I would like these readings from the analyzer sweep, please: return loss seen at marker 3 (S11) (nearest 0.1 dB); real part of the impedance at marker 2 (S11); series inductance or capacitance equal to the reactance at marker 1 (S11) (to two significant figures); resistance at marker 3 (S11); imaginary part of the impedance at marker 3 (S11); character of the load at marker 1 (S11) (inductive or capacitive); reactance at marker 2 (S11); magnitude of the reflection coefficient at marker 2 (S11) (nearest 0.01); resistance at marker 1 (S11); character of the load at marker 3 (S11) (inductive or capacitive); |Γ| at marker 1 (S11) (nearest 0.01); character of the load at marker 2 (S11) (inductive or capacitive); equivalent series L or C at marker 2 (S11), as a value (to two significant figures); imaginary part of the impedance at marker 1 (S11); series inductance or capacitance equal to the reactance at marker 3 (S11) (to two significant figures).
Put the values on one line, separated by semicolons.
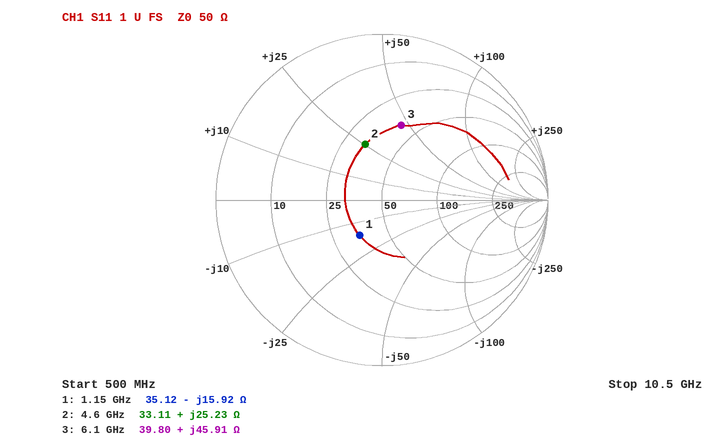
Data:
6.6 dB; 33.11 Ω; 8.7 pF; 39.80 Ω; +45.91 Ω; capacitive; +25.23 Ω; 0.35; 35.12 Ω; inductive; 0.25; inductive; 870 pH; -15.92 Ω; 1.2 nH
